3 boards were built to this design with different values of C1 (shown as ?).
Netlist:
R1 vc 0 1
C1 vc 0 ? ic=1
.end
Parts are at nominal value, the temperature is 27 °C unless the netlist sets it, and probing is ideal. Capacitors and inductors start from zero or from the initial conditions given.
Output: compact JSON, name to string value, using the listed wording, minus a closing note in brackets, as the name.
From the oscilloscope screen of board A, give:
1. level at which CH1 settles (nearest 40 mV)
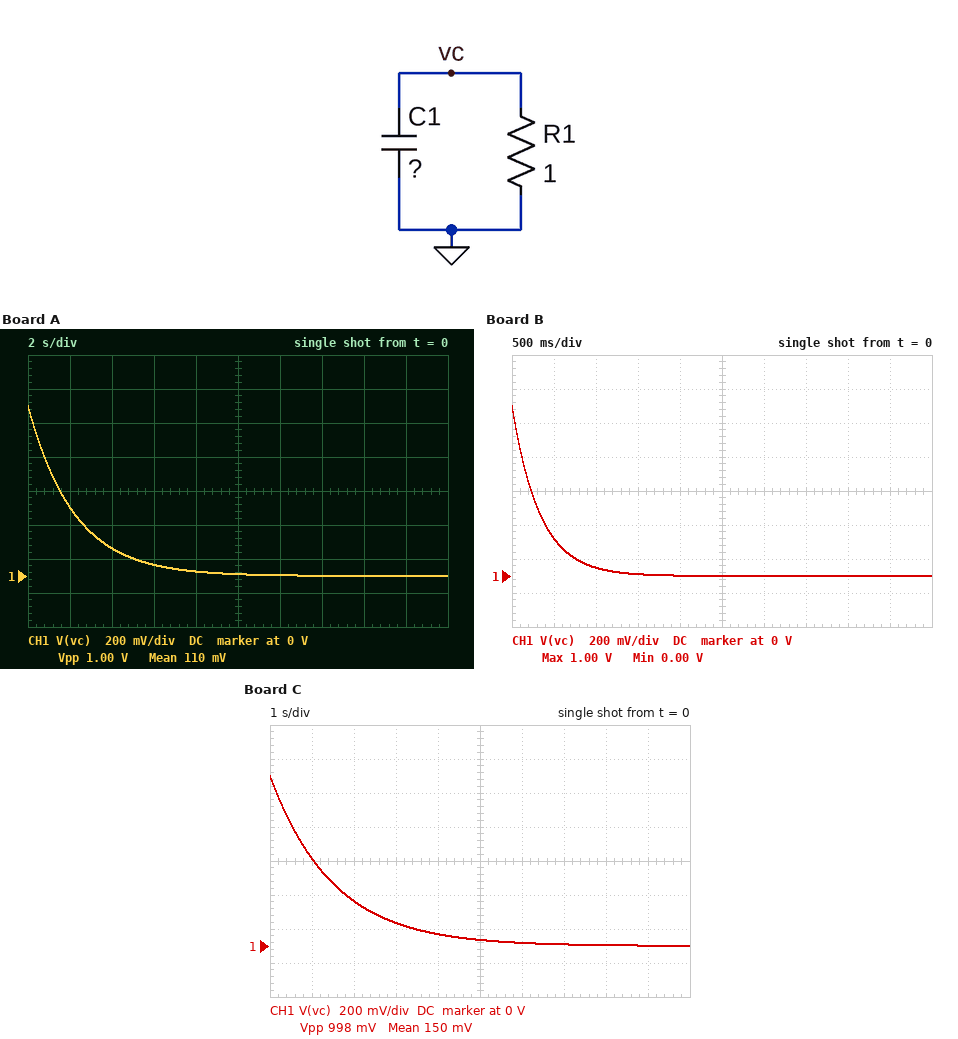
{"level at which CH1 settles": "0 V"}
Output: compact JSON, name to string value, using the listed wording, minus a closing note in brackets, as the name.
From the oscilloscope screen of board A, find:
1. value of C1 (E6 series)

{"value of C1": "2.2 F"}
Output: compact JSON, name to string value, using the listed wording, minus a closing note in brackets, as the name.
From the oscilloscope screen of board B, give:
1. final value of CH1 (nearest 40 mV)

{"final value of CH1": "0 V"}
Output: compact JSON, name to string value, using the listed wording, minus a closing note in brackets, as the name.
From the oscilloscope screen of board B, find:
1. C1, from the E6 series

{"C1, from the E6 series": "330 mF"}
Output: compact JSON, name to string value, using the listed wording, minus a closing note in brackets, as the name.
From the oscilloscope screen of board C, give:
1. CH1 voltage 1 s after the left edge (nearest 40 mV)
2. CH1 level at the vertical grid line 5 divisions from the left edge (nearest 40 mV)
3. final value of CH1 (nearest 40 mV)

{"CH1 voltage 1 s after the left edge": "520 mV", "CH1 level at the vertical grid line 5 divisions from the left edge": "40 mV", "final value of CH1": "0 V"}
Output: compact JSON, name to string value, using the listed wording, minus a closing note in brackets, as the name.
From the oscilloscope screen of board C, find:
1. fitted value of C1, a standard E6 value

{"fitted value of C1, a standard E6 value": "1.5 F"}
